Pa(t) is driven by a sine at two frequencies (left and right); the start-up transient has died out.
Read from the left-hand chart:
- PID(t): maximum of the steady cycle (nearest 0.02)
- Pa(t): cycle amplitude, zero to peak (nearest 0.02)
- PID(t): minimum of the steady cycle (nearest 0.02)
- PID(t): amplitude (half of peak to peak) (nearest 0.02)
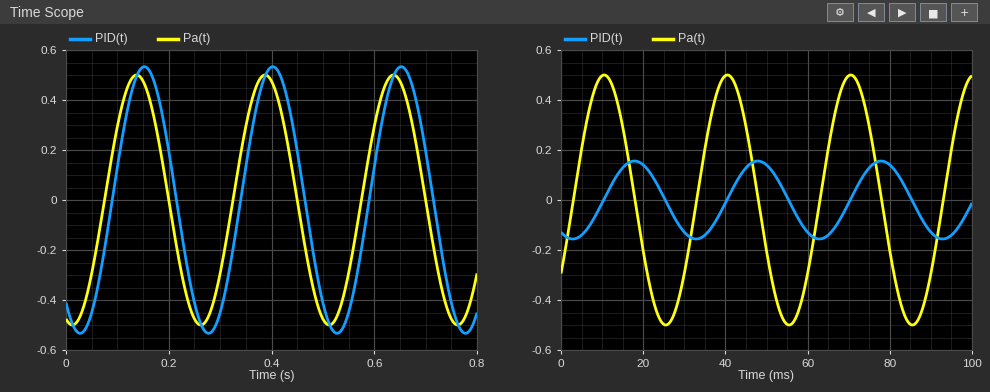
0.54
0.50
-0.54
0.54
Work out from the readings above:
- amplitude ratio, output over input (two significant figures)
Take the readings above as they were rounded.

1.1
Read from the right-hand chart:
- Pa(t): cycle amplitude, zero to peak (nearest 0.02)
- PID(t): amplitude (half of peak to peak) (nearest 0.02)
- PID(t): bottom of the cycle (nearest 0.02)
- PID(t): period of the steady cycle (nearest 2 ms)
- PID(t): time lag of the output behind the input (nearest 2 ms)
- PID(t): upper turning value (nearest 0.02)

0.50
0.16
-0.16
30 ms
8 ms
0.16
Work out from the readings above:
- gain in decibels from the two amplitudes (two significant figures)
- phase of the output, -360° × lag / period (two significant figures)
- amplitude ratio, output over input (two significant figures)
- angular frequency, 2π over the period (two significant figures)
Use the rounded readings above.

-9.9 dB
-96°
0.32
0.21 rad/ms
